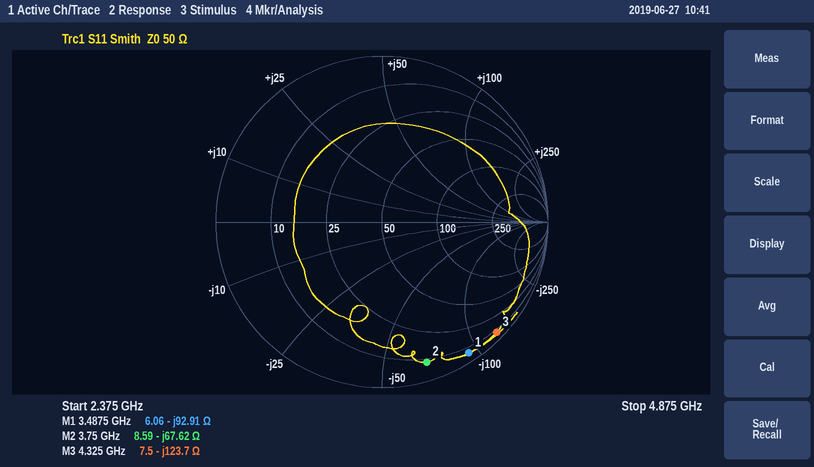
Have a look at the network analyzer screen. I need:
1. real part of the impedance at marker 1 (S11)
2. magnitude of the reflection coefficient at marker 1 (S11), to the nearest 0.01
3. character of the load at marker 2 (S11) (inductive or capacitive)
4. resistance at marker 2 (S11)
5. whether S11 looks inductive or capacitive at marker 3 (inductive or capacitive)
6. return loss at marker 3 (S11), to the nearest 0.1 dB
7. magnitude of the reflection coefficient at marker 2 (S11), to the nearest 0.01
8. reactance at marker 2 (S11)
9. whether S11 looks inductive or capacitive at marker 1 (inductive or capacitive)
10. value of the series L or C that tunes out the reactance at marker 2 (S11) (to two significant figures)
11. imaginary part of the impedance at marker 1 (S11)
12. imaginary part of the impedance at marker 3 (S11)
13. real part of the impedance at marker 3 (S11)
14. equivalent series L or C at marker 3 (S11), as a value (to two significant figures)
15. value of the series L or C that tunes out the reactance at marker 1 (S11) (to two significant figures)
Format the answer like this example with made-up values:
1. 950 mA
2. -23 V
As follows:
1. 6.06 Ω
2. 0.95
3. capacitive
4. 8.59 Ω
5. capacitive
6. 0.4 dB
7. 0.89
8. -67.62 Ω
9. capacitive
10. 2.9 nH
11. -92.91 Ω
12. -123.7 Ω
13. 7.5 Ω
14. 300 fF
15. 4.2 nH
